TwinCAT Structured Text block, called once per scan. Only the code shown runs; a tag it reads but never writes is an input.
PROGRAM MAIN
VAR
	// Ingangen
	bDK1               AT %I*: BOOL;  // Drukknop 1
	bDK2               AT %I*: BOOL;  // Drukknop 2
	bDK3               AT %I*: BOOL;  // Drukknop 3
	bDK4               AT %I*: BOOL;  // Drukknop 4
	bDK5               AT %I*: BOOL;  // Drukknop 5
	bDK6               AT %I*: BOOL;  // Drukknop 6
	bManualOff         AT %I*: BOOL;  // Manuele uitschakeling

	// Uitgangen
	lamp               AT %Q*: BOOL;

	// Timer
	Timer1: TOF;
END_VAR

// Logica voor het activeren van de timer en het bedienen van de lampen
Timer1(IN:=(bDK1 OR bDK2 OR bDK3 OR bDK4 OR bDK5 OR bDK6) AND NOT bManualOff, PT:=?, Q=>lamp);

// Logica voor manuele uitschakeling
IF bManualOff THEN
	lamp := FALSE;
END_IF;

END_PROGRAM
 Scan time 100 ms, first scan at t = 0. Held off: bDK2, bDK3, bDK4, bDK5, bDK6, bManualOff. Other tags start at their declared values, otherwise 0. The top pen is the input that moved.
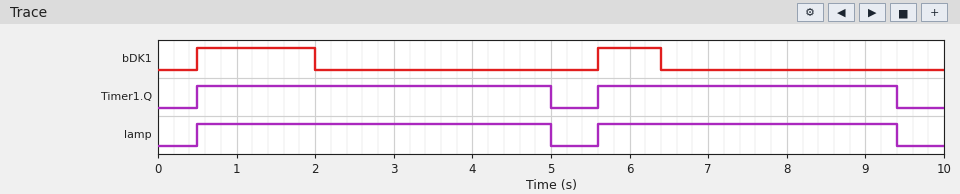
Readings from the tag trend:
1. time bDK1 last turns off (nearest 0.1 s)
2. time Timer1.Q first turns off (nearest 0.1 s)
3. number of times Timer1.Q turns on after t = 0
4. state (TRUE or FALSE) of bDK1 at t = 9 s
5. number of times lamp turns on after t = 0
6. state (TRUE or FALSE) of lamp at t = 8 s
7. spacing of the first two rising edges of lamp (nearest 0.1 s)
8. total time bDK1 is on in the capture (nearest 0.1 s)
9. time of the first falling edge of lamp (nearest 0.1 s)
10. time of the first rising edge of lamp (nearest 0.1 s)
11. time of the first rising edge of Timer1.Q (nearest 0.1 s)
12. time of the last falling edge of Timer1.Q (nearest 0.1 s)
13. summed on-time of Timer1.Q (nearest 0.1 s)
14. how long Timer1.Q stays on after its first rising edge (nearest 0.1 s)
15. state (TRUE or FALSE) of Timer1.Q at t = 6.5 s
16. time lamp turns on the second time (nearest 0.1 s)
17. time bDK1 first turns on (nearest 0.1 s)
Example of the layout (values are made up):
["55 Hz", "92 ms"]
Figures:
["6.4 s", "5.0 s", "2", "FALSE", "2", "TRUE", "5.1 s", "2.3 s", "5.0 s", "0.5 s", "0.5 s", "9.4 s", "8.3 s", "4.5 s", "TRUE", "5.6 s", "0.5 s"]
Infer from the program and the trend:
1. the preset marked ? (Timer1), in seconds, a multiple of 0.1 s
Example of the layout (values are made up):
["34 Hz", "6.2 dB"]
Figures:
["3.0 s"]
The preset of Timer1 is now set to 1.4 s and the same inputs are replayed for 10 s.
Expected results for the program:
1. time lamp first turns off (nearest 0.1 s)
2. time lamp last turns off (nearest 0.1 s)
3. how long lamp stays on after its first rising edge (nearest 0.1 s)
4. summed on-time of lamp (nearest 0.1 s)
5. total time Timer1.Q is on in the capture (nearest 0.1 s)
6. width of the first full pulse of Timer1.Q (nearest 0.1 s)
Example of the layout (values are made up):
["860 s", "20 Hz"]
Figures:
["3.4 s", "7.8 s", "2.9 s", "5.1 s", "5.1 s", "2.9 s"]
